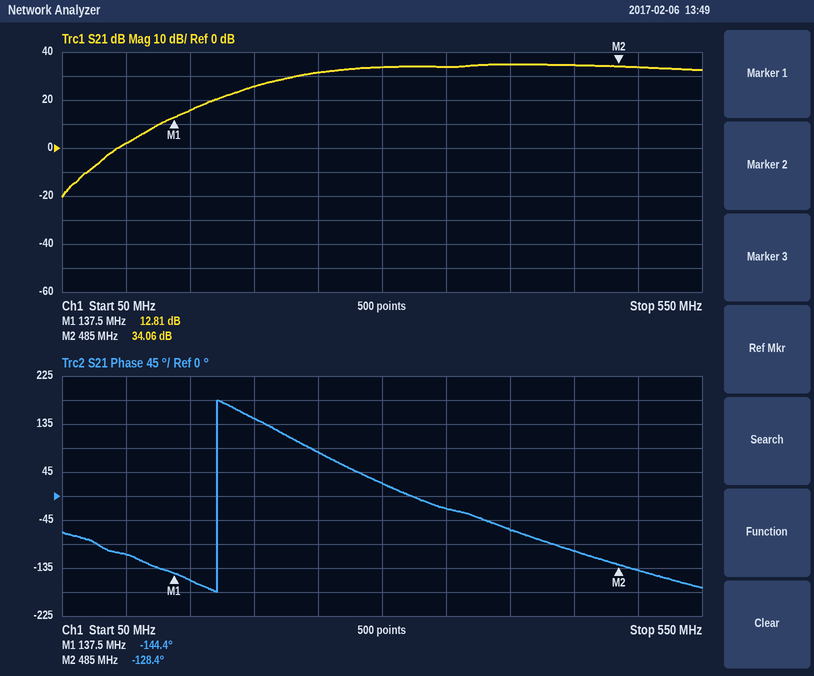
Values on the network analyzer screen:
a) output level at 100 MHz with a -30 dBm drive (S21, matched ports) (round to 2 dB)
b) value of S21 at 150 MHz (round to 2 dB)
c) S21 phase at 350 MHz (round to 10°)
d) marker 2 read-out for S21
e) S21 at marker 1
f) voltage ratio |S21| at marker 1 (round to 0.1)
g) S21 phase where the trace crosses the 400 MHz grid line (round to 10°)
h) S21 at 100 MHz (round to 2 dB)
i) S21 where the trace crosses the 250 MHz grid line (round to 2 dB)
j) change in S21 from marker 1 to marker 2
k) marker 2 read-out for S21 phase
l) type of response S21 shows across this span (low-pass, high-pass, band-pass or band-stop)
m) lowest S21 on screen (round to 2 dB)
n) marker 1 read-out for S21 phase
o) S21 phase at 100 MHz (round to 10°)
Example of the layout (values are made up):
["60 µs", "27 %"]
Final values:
["-28 dBm", "16 dB", "-20°", "34.06 dB", "12.81 dB", "4.4", "-60°", "2 dB", "32 dB", "21.25 dB", "-128.4°", "high-pass", "-20 dB", "-144.4°", "-110°"]
